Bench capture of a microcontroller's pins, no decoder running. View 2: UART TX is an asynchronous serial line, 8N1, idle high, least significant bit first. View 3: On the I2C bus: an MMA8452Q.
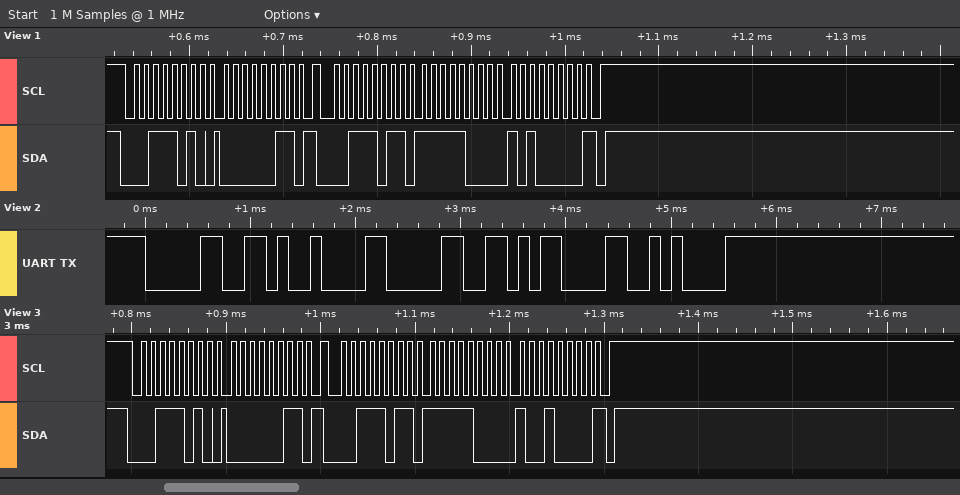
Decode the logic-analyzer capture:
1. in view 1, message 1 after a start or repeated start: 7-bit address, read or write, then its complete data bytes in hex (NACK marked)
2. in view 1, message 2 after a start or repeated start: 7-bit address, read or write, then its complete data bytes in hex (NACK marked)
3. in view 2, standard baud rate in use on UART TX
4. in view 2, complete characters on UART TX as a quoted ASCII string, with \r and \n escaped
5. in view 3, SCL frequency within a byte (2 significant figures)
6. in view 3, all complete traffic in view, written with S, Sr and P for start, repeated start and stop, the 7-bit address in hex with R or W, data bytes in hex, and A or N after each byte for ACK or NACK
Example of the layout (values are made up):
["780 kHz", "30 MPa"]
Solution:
["0x1D write: 03", "0x1D read: F8 A0 NACK", "9600 baud", "\"0\\t0\\r\\n\"", "100 kHz", "S 1DW A 03 A Sr 1DR A F8 A 90 N P"]
